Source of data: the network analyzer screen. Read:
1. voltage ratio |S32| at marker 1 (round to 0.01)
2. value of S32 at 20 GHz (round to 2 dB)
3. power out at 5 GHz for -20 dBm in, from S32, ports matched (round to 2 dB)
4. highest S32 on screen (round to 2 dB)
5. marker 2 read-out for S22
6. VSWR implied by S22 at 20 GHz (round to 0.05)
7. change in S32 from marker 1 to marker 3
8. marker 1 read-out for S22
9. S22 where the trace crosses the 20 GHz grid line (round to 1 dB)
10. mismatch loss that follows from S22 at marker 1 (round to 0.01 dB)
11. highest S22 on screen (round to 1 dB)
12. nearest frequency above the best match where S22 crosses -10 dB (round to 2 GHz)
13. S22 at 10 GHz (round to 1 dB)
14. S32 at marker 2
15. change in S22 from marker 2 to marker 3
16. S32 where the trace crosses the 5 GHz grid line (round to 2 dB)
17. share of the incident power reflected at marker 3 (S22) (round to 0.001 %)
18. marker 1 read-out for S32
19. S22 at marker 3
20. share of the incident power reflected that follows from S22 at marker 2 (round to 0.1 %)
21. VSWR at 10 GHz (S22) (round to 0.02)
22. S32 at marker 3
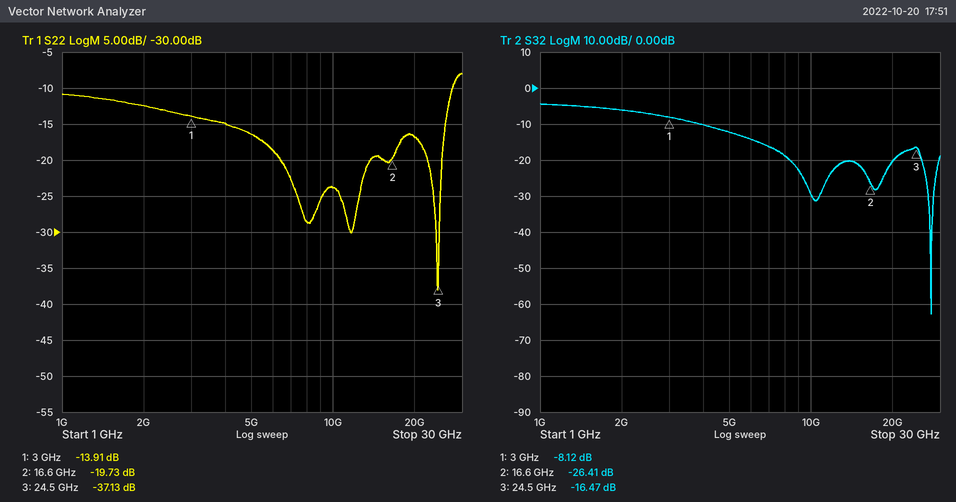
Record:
0.39
-20 dB
-32 dBm
-4 dB
-19.73 dB
1.35
-8.35 dB
-13.91 dB
-17 dB
0.18 dB
-8 dB
28 GHz
-24 dB
-26.41 dB
-17.40 dB
-12 dB
0.019 %
-8.12 dB
-37.13 dB
1.1 %
1.14
-16.47 dB
